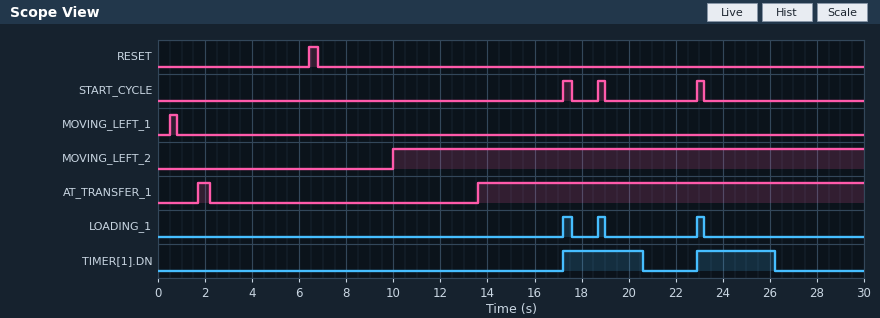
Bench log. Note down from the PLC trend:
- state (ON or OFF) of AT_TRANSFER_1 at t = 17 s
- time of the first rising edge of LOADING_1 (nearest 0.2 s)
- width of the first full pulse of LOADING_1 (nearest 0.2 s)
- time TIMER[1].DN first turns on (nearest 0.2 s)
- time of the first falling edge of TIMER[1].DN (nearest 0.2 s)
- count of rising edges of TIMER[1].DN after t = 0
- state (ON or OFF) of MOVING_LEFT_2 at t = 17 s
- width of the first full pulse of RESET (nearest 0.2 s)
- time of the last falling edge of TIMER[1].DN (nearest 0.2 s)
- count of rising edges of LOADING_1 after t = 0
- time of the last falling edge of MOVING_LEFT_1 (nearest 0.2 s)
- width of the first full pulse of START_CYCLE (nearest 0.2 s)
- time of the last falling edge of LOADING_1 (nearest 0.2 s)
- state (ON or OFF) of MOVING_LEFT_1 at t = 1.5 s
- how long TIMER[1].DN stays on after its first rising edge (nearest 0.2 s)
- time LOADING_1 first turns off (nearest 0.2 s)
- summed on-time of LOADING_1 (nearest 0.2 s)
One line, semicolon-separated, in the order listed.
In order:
ON; 17.2 s; 0.4 s; 17.2 s; 20.6 s; 2; ON; 0.4 s; 26.2 s; 3; 0.8 s; 0.4 s; 23.2 s; OFF; 3.4 s; 17.6 s; 1.0 s
